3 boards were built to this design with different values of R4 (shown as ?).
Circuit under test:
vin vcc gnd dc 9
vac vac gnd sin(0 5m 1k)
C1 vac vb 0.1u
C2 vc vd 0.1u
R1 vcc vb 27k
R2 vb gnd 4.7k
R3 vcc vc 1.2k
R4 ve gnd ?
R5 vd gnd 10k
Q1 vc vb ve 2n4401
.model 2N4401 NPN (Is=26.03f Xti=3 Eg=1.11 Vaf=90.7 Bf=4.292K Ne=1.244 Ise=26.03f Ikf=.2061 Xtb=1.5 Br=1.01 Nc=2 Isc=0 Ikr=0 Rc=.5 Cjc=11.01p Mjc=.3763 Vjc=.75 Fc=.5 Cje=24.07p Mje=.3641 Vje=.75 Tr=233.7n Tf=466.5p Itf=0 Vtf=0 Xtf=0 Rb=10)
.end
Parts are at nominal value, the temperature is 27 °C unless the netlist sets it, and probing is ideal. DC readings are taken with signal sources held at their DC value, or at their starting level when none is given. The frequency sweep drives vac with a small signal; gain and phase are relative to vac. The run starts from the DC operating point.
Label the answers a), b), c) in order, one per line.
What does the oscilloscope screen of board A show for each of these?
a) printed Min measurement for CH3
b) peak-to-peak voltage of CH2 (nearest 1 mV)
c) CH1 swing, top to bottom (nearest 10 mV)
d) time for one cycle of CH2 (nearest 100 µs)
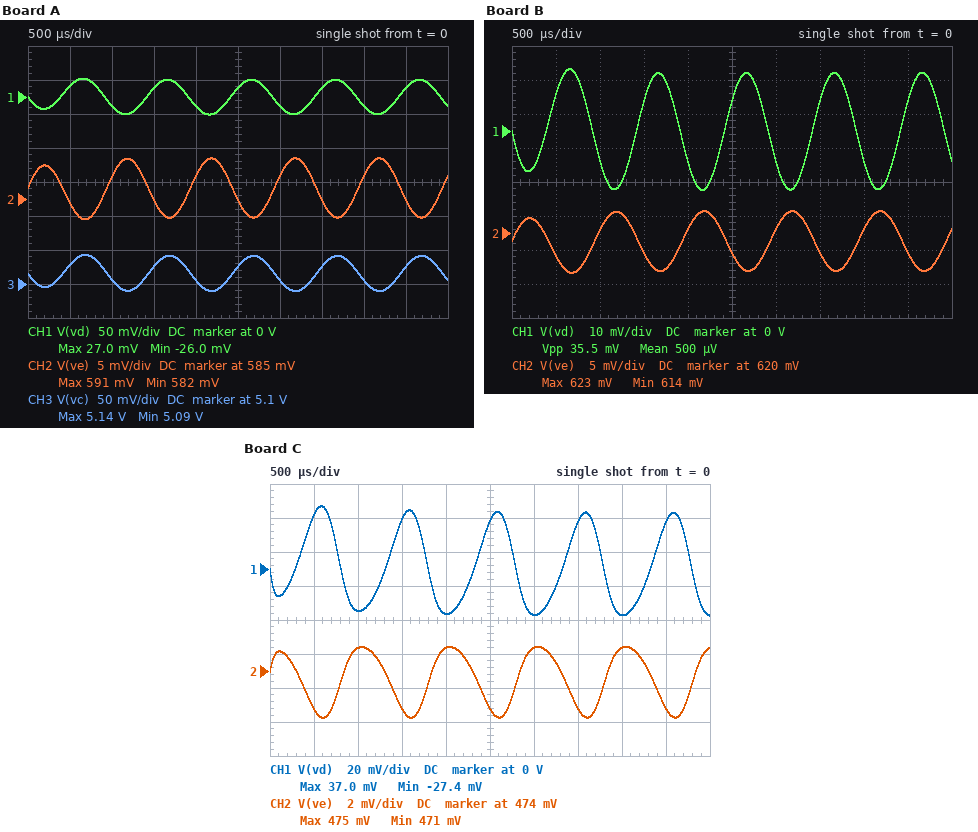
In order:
a) 5.09 V
b) 9 mV
c) 50 mV
d) 1.0 ms
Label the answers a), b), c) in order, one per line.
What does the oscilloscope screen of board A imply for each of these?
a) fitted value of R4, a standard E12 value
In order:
a) 180 Ω
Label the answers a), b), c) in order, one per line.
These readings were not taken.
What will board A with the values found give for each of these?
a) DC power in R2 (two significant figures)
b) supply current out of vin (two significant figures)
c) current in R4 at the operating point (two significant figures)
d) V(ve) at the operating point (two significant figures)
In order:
a) 330 µW
b) 3.5 mA
c) 3.3 mA
d) 590 mV
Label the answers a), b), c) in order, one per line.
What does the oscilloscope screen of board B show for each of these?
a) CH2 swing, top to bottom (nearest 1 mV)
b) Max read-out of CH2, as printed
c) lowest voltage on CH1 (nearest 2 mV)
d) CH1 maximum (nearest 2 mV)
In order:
a) 9 mV
b) 623 mV
c) -18 mV
d) 18 mV
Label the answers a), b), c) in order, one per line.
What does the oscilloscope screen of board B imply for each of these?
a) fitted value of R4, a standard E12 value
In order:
a) 270 Ω
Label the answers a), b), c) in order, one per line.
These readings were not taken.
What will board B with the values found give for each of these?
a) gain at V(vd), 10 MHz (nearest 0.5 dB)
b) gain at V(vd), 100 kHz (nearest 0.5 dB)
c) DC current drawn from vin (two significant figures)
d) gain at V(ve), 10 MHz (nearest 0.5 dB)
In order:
a) 11.0 dB
b) 11.5 dB
c) 2.6 mA
d) -0.5 dB
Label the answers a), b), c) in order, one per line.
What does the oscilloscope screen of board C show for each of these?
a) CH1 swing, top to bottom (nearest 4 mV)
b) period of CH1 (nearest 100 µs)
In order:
a) 64 mV
b) 1.0 ms
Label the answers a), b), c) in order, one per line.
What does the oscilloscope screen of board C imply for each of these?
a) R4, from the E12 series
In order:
a) 68 Ω
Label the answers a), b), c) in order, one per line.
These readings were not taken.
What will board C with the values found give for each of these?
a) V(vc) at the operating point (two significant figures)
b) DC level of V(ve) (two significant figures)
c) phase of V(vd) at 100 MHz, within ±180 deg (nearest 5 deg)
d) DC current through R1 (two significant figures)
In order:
a) 690 mV
b) 470 mV
c) 30 deg
d) 290 µA
